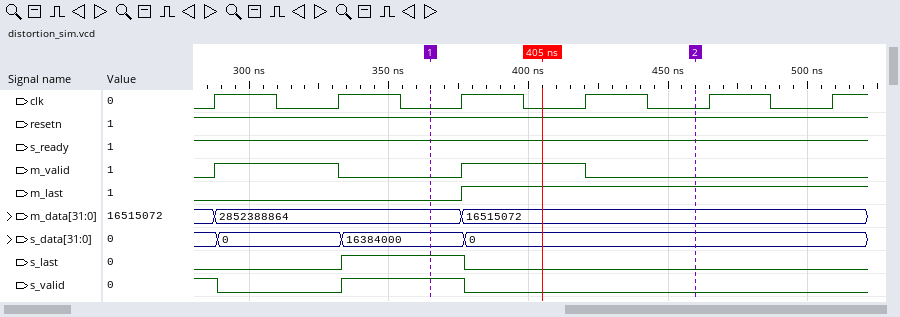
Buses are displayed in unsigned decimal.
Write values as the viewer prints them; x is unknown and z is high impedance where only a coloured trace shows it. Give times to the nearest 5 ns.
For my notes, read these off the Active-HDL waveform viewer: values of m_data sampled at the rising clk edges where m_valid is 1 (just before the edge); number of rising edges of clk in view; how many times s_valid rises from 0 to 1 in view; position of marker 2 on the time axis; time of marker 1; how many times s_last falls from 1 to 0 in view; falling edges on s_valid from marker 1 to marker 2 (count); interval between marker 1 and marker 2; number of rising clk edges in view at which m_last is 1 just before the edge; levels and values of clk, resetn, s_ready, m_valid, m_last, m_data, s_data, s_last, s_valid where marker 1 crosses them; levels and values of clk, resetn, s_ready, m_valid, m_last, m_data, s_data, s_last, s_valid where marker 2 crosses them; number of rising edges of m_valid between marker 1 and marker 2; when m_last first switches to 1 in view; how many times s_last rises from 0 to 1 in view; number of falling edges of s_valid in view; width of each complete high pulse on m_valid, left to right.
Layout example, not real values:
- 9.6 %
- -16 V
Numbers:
- 2852388864, 16515072
- 6
- 1
- 460 ns
- 365 ns
- 1
- 1
- 95 ns
- 3
- clk=0, resetn=1, s_ready=1, m_valid=0, m_last=0, m_data=2852388864, s_data=16384000, s_last=1, s_valid=1
- clk=0, resetn=1, s_ready=1, m_valid=0, m_last=1, m_data=16515072, s_data=0, s_last=0, s_valid=0
- 1
- 375 ns
- 1
- 2
- 45 ns, 45 ns
